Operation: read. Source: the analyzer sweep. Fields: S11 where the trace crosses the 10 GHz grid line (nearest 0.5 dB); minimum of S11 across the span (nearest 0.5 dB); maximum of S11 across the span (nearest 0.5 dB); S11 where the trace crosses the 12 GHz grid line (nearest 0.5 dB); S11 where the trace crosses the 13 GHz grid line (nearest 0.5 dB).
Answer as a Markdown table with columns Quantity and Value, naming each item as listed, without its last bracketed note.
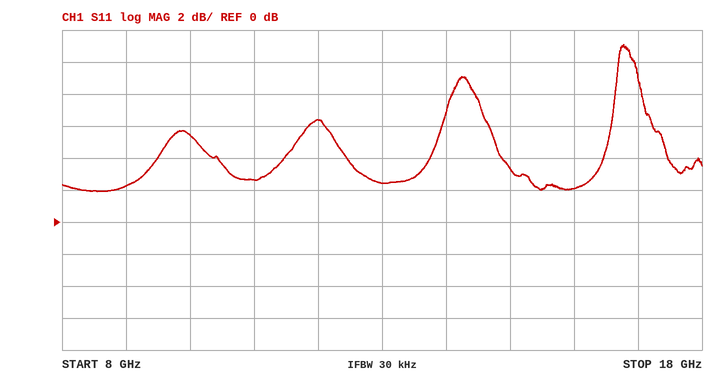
| Quantity | Value |
|---|---|
| S11 where the trace crosses the 10 GHz grid line | 5.5 dB |
| minimum of S11 across the span | 2.0 dB |
| maximum of S11 across the span | 11.0 dB |
| S11 where the trace crosses the 12 GHz grid line | 6.5 dB |
| S11 where the trace crosses the 13 GHz grid line | 2.5 dB |
